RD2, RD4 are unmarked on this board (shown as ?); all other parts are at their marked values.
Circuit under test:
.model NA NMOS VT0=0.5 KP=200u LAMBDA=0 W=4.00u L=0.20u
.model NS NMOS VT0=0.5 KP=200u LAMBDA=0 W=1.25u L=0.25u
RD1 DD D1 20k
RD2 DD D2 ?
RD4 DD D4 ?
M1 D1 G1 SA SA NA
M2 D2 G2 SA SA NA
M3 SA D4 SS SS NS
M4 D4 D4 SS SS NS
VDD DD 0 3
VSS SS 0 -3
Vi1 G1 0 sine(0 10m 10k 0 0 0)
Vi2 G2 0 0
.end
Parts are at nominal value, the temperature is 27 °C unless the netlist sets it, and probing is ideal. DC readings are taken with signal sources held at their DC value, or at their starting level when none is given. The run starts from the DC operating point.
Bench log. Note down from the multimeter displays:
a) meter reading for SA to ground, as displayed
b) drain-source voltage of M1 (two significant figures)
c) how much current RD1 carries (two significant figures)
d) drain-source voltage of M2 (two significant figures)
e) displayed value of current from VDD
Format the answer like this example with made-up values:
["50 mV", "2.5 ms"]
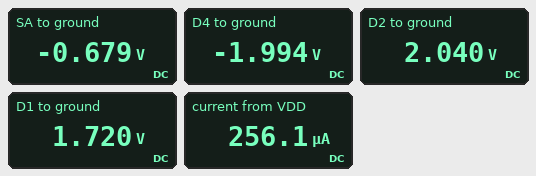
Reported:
["-0.679 V", "2.4 V", "64 µA", "2.7 V", "256.1 µA"]
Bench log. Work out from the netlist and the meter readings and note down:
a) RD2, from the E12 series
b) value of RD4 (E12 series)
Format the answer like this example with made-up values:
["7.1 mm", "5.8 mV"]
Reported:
["15 kΩ", "39 kΩ"]
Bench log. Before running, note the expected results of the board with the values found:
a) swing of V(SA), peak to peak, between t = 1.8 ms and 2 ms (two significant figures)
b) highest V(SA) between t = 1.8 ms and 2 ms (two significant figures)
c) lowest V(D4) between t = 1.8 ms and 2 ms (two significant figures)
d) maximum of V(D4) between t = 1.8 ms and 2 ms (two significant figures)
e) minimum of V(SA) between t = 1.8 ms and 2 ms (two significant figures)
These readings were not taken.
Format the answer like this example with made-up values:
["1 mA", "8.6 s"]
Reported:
["10 mV", "-670 mV", "-2.0 V", "-2.0 V", "-680 mV"]
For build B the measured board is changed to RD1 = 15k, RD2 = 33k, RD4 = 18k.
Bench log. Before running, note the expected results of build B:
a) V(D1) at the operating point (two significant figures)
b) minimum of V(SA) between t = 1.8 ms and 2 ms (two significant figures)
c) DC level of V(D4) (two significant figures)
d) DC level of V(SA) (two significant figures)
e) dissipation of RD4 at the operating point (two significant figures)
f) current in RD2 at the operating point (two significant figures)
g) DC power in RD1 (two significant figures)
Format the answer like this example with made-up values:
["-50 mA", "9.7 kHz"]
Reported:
["680 mV", "-790 mV", "-1.8 V", "-780 mV", "1.3 mW", "110 µA", "360 µW"]
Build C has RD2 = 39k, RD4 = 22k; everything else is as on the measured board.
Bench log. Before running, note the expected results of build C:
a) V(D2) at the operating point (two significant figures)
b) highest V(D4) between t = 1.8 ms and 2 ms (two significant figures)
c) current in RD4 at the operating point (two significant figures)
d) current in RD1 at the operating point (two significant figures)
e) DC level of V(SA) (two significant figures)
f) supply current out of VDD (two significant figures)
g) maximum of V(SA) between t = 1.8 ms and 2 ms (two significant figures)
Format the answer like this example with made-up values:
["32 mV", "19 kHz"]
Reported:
["-630 mV", "-1.8 V", "220 µA", "130 µA", "-750 mV", "440 µA", "-740 mV"]
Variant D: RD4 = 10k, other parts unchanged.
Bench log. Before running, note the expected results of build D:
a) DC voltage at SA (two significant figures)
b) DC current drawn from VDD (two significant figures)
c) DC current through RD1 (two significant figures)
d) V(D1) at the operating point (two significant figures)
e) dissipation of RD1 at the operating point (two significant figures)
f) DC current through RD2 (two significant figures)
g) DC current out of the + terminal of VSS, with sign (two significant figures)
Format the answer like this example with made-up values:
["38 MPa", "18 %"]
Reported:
["-1.0 V", "910 µA", "200 µA", "-920 mV", "770 µW", "260 µA", "-910 µA"]
